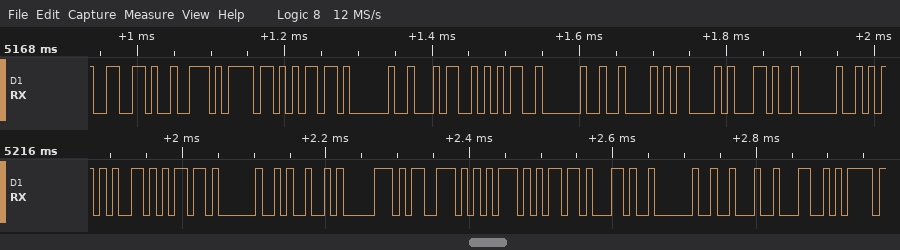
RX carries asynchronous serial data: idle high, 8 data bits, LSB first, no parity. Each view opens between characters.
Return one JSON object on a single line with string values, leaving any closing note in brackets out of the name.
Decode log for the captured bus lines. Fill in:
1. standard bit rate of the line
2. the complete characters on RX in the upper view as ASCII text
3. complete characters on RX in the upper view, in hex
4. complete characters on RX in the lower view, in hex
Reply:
{"standard bit rate of the line": "115200 baud", "the complete characters on RX in the upper view as ASCII text": "\"from 45 BC, \"", "complete characters on RX in the upper view, in hex": "66, 72, 6F, 6D, 20, 34, 35, 20, 42, 43, 2C, 20", "complete characters on RX in the lower view, in hex": "65, 6D, 20, 49, 70, 73, 75, 6D, 2C, 20, 22, 4C"}
